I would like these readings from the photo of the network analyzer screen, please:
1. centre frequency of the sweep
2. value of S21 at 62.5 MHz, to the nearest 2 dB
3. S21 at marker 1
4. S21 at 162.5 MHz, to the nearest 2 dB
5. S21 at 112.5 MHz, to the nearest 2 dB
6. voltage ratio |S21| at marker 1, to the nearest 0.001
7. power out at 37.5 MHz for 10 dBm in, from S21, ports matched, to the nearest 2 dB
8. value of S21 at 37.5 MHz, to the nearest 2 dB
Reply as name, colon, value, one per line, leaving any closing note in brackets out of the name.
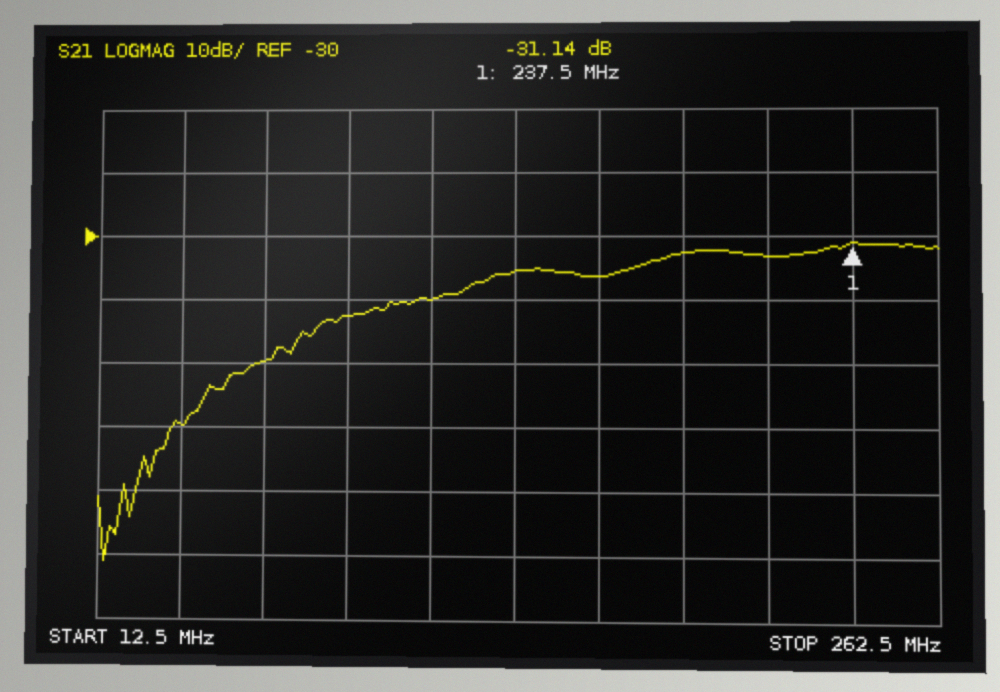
centre frequency of the sweep: 137.5 MHz
value of S21 at 62.5 MHz, to the nearest 2 dB: -50 dB
S21 at marker 1: -31.14 dB
S21 at 162.5 MHz, to the nearest 2 dB: -36 dB
S21 at 112.5 MHz, to the nearest 2 dB: -40 dB
voltage ratio |S21| at marker 1, to the nearest 0.001: 0.028
power out at 37.5 MHz for 10 dBm in, from S21, ports matched, to the nearest 2 dB: -50 dBm
value of S21 at 37.5 MHz, to the nearest 2 dB: -60 dB
